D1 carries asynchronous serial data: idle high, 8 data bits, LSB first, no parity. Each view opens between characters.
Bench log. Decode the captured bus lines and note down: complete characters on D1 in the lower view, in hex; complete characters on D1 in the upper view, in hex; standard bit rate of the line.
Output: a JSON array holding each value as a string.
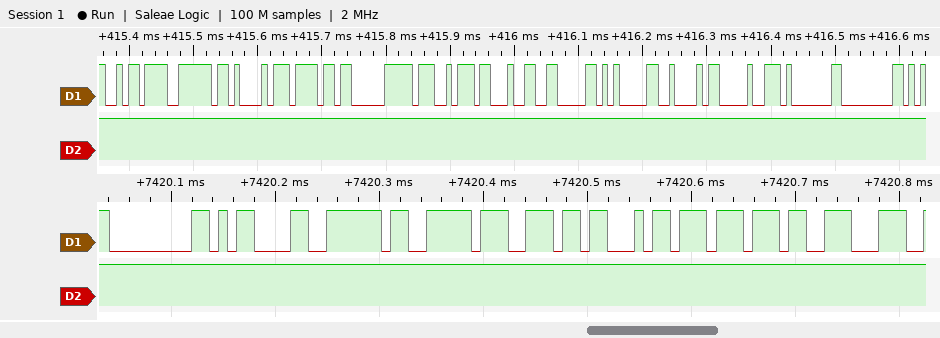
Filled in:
["00, 0D, 7E, BE, 6E, B4, 77, 8E", "DA, 7E, A1, 6F, E0, A7, 23, 06, 05, 42, 90, 01, 00", "115200 baud"]
